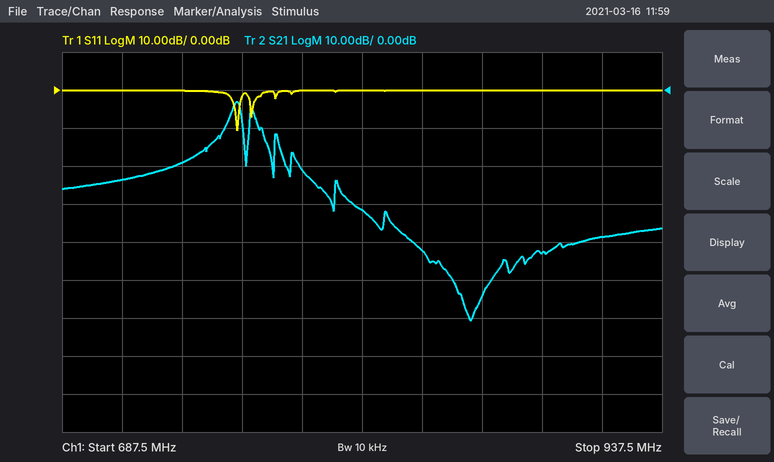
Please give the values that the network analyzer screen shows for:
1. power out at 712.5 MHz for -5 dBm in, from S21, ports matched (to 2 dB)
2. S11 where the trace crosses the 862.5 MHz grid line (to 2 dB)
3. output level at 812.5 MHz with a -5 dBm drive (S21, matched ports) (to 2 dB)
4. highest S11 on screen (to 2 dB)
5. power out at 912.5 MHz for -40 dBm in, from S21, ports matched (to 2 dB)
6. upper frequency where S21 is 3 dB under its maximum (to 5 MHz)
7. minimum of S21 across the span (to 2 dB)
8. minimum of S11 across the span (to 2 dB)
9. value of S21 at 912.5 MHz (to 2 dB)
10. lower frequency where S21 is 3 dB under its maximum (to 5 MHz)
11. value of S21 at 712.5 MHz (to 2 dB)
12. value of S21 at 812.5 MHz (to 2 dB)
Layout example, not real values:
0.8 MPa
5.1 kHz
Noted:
-28 dBm
0 dB
-36 dBm
0 dB
-78 dBm
760 MHz
-60 dB
-10 dB
-38 dB
760 MHz
-24 dB
-32 dB
